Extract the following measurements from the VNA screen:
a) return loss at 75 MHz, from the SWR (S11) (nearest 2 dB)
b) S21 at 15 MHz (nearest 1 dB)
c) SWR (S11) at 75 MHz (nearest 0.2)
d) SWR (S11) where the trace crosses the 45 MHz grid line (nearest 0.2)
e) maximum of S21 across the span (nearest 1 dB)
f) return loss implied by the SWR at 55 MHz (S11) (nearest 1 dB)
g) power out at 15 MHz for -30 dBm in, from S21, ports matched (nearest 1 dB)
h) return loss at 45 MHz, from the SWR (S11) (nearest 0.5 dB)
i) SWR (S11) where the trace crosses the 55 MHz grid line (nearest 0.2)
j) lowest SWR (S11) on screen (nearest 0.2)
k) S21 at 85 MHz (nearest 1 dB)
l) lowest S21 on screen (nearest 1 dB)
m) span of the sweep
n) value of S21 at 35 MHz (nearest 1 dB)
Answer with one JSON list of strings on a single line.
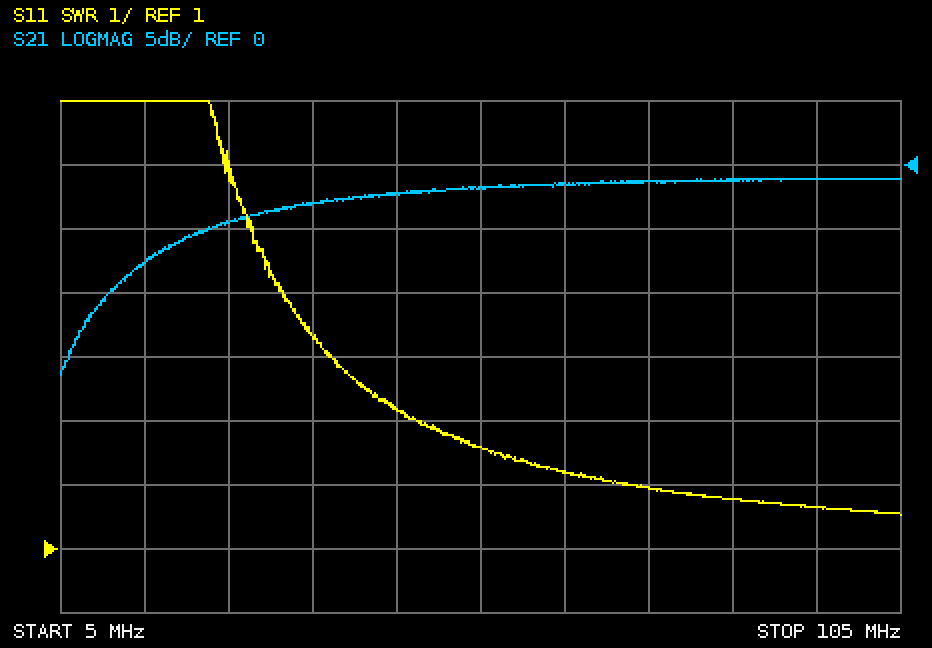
["10 dB", "-8 dB", "2.0", "3.2", "-1 dB", "7 dB", "-38 dBm", "5.5 dB", "2.6", "1.6", "-1 dB", "-16 dB", "100 MHz", "-3 dB"]
